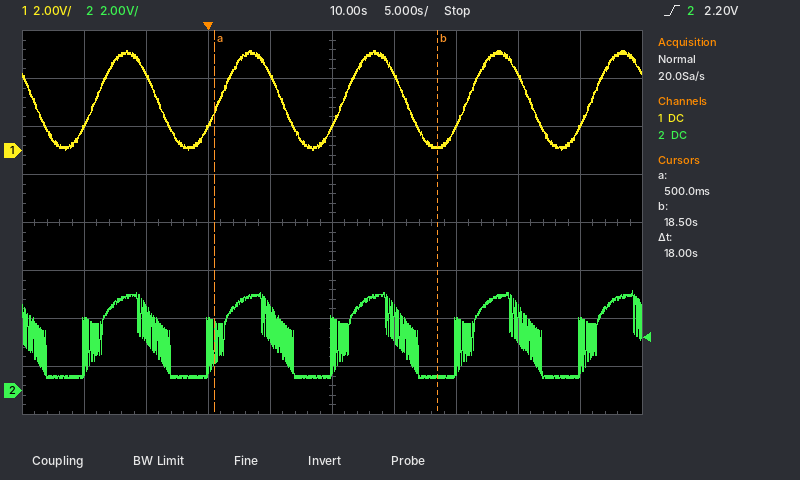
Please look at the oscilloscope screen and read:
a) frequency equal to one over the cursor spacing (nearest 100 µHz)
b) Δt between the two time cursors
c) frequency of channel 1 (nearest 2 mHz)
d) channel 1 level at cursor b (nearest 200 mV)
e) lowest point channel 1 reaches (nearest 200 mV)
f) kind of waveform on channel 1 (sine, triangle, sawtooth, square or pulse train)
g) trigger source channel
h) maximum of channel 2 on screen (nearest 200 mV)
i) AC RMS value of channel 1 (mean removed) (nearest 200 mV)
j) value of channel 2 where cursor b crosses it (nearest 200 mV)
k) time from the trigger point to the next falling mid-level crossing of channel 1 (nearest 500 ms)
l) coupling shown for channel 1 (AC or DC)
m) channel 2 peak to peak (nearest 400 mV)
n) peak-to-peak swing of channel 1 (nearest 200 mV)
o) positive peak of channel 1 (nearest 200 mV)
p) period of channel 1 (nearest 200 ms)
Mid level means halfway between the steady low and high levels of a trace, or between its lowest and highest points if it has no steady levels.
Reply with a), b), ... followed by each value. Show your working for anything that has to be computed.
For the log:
a) 1 / 18 s ≈ 55.6 mHz
b) 18 s
c) 1 / 10.0 s ≈ 100 mHz
d) 200 mV
e) 0.0 V
f) sine
g) channel 2
h) 4.2 V
i) 4.2 V / (2√2) ≈ 1.48 V, so 1.4 V to the nearest 200 mV
j) 600 mV
k) 6.0 s
l) DC
m) 3.6 V
n) 4.2 V − (0.0 V) = 4.2 V
o) 4.2 V
p) 10.0 s
